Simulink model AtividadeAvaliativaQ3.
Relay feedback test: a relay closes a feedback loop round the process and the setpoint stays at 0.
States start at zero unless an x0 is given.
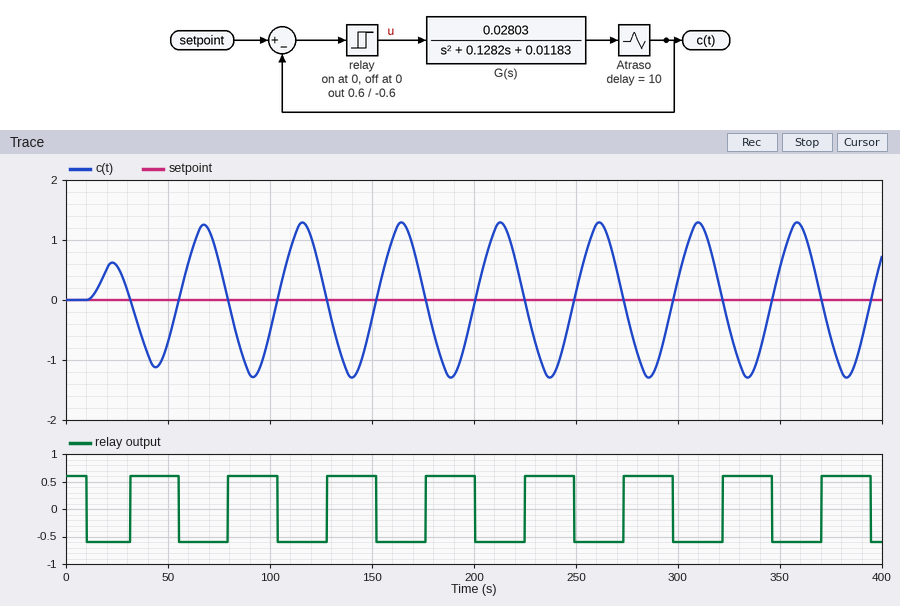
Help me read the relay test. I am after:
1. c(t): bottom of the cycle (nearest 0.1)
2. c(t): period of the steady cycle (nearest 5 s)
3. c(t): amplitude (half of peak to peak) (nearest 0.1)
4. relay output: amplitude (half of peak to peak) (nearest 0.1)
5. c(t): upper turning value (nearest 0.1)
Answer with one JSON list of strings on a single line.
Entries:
["-1.3", "50 s", "1.3", "0.6", "1.3"]
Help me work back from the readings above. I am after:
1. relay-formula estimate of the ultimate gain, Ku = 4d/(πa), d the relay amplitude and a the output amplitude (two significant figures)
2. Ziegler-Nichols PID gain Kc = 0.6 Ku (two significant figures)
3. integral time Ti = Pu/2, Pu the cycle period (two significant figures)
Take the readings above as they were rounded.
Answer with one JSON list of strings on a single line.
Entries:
["0.59", "0.35", "25 s"]
